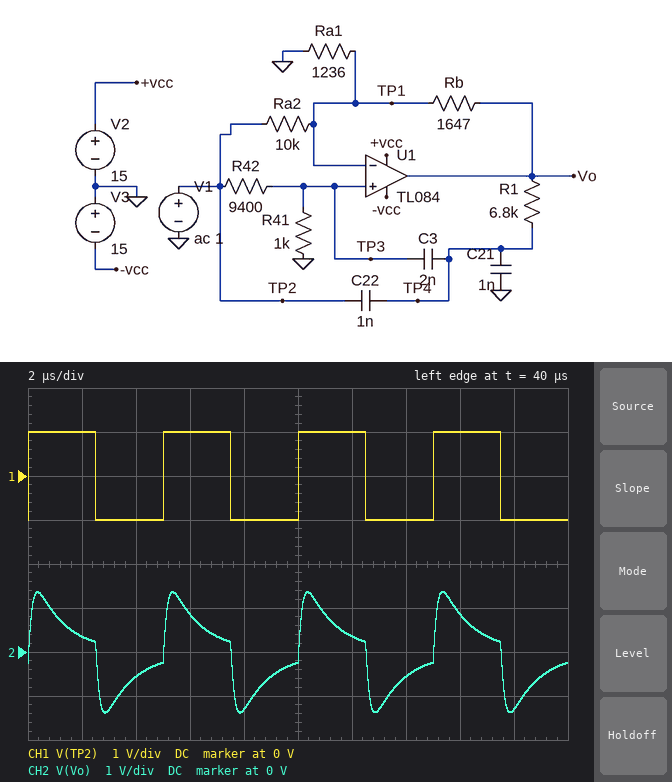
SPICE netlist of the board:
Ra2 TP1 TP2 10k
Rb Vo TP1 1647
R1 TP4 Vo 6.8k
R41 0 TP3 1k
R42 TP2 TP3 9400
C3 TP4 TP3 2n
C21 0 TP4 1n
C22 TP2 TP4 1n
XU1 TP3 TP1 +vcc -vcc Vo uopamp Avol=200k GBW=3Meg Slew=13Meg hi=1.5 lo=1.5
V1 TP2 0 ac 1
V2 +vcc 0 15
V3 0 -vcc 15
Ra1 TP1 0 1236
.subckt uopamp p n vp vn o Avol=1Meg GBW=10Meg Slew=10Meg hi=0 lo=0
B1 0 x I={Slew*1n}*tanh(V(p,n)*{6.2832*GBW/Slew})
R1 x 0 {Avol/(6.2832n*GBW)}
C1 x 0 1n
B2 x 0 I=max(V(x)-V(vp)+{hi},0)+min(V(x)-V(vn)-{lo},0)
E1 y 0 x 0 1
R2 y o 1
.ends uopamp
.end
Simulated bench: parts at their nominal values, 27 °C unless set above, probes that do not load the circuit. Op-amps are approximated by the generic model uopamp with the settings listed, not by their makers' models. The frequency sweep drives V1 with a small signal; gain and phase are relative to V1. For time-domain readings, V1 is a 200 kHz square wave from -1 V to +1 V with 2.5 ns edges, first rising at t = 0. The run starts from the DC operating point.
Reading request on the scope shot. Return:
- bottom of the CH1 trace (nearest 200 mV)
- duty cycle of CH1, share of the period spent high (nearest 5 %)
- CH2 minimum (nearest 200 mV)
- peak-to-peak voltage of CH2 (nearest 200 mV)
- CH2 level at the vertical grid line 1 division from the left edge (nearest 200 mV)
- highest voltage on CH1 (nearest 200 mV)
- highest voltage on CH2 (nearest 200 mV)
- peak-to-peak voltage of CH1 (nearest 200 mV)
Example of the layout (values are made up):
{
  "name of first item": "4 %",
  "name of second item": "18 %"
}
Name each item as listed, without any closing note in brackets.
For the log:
{
  "bottom of the CH1 trace": "-1.0 V",
  "duty cycle of CH1, share of the period spent high": "50 %",
  "CH2 minimum": "-1.4 V",
  "peak-to-peak voltage of CH2": "2.8 V",
  "CH2 level at the vertical grid line 1 division from the left edge": "400 mV",
  "highest voltage on CH1": "1.0 V",
  "highest voltage on CH2": "1.4 V",
  "peak-to-peak voltage of CH1": "2.0 V"
}
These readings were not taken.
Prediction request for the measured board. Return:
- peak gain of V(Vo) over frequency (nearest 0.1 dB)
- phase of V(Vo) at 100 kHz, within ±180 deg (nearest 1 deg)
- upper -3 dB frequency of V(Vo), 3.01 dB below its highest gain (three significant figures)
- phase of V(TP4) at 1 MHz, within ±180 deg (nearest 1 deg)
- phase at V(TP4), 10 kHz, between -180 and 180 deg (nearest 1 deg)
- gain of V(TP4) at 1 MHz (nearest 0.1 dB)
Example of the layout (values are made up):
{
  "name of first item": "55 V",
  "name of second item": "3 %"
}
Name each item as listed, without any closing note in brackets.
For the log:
{
  "peak gain of V(Vo) over frequency": "-0.5 dB",
  "phase of V(Vo) at 100 kHz, within ±180 deg": "49 deg",
  "upper -3 dB frequency of V(Vo), 3.01 dB below its highest gain": "1.50 MHz",
  "phase of V(TP4) at 1 MHz, within ±180 deg": "4 deg",
  "phase at V(TP4), 10 kHz, between -180 and 180 deg": "27 deg",
  "gain of V(TP4) at 1 MHz": "-6.2 dB"
}
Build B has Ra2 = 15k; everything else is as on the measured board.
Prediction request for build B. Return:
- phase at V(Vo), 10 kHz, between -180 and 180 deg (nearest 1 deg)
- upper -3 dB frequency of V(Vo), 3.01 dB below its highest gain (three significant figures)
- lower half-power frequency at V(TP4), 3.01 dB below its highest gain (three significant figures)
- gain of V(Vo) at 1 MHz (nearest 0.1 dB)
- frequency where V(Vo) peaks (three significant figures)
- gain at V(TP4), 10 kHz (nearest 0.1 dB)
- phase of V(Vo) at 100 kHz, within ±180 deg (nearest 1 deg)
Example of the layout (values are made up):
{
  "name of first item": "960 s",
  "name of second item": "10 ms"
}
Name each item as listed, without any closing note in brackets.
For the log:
{
  "phase at V(Vo), 10 kHz, between -180 and 180 deg": "25 deg",
  "upper -3 dB frequency of V(Vo), 3.01 dB below its highest gain": "1.53 MHz",
  "lower half-power frequency at V(TP4), 3.01 dB below its highest gain": "61.6 kHz",
  "gain of V(Vo) at 1 MHz": "-1.5 dB",
  "frequency where V(Vo) peaks": "432 kHz",
  "gain at V(TP4), 10 kHz": "-11.0 dB",
  "phase of V(Vo) at 100 kHz, within ±180 deg": "45 deg"
}
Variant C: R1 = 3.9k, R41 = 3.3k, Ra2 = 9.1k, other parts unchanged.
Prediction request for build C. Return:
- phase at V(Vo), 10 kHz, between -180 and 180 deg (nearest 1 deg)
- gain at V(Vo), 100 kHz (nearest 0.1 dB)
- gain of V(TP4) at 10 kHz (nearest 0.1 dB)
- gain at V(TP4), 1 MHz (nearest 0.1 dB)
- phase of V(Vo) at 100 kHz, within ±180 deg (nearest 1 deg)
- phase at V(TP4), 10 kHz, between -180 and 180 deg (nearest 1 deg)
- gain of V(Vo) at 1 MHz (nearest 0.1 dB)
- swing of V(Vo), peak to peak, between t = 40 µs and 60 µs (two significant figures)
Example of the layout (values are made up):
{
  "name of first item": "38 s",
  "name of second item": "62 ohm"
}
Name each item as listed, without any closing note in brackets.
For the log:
{
  "phase at V(Vo), 10 kHz, between -180 and 180 deg": "21 deg",
  "gain at V(Vo), 100 kHz": "0.3 dB",
  "gain of V(TP4) at 10 kHz": "-5.8 dB",
  "gain at V(TP4), 1 MHz": "-6.2 dB",
  "phase of V(Vo) at 100 kHz, within ±180 deg": "0 deg",
  "phase at V(TP4), 10 kHz, between -180 and 180 deg": "7 deg",
  "gain of V(Vo) at 1 MHz": "-1.9 dB",
  "swing of V(Vo), peak to peak, between t = 40 µs and 60 µs": "2.1 V"
}
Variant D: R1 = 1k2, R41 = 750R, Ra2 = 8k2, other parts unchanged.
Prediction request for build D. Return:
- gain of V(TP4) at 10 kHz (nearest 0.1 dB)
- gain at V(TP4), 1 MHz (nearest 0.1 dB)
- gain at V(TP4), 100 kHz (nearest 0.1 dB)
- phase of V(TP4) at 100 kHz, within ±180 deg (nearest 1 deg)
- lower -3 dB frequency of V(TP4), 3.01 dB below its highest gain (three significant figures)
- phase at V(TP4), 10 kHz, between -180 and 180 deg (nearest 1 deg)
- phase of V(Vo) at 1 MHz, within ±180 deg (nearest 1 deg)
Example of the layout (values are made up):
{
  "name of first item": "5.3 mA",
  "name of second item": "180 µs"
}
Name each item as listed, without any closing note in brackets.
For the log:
{
  "gain of V(TP4) at 10 kHz": "-22.8 dB",
  "gain at V(TP4), 1 MHz": "-6.6 dB",
  "gain at V(TP4), 100 kHz": "-5.2 dB",
  "phase of V(TP4) at 100 kHz, within ±180 deg": "28 deg",
  "lower -3 dB frequency of V(TP4), 3.01 dB below its highest gain": "52.5 kHz",
  "phase at V(TP4), 10 kHz, between -180 and 180 deg": "97 deg",
  "phase of V(Vo) at 1 MHz, within ±180 deg": "-29 deg"
}
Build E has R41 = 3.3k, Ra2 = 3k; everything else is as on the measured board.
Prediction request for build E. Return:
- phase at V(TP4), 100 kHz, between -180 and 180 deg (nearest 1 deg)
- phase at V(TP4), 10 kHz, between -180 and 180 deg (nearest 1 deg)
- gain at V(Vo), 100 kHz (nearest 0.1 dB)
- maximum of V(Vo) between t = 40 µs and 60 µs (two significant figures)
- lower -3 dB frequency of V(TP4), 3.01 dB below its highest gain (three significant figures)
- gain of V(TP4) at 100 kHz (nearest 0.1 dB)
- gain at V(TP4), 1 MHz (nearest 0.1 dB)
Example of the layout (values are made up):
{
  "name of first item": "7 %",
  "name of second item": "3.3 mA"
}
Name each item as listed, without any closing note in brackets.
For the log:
{
  "phase at V(TP4), 100 kHz, between -180 and 180 deg": "3 deg",
  "phase at V(TP4), 10 kHz, between -180 and 180 deg": "25 deg",
  "gain at V(Vo), 100 kHz": "-1.8 dB",
  "maximum of V(Vo) between t = 40 µs and 60 µs": "950 mV",
  "lower -3 dB frequency of V(TP4), 3.01 dB below its highest gain": "9.63 kHz",
  "gain of V(TP4) at 100 kHz": "-6.2 dB",
  "gain at V(TP4), 1 MHz": "-6.1 dB"
}
